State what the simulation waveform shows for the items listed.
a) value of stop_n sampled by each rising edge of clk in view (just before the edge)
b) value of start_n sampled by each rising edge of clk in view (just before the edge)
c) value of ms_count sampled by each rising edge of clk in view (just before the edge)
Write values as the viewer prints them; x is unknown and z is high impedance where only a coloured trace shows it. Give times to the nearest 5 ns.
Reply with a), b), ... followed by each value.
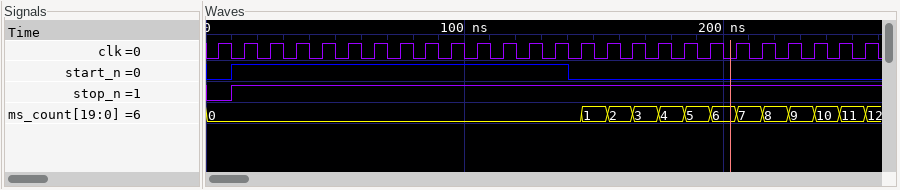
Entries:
a) 0 1 1 1 1 1 1 1 1 1 1 1 1 1 1 1 1 1 1 1 1 1 1 1 1 1
b) 0 1 1 1 1 1 1 1 1 1 1 1 1 1 0 0 0 0 0 0 0 0 0 0 0 0
c) 0, 0, 0, 0, 0, 0, 0, 0, 0, 0, 0, 0, 0, 0, 0, 1, 2, 3, 4, 5, 6, 7, 8, 9, 10, 11
